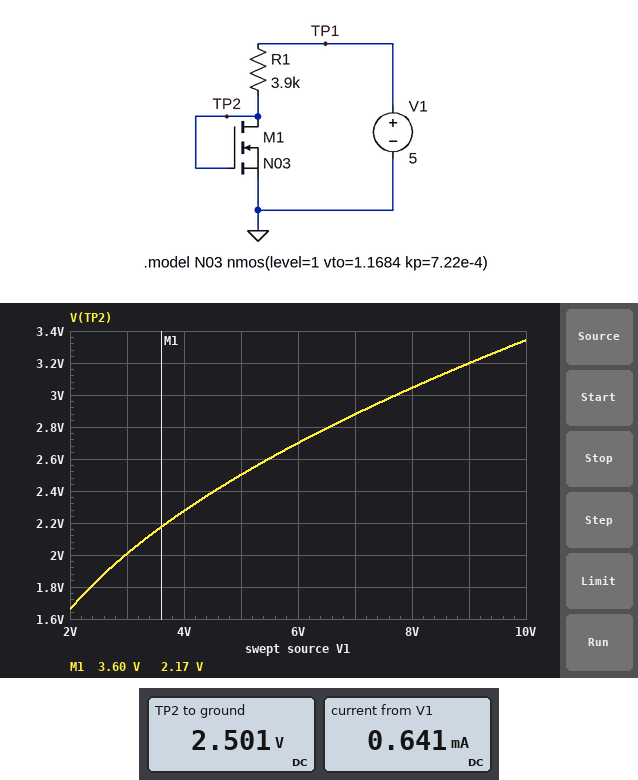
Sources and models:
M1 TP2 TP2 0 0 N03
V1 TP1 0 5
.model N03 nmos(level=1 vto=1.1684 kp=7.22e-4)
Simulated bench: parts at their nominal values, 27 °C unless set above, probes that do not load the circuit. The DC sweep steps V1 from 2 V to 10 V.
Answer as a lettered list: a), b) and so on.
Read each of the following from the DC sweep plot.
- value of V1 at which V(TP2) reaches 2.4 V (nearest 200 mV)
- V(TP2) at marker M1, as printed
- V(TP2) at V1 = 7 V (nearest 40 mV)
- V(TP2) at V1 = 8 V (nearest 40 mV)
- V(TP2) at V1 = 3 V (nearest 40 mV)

a) 4.6 V
b) 2.17 V
c) 2.88 V
d) 3.04 V
e) 2.00 V
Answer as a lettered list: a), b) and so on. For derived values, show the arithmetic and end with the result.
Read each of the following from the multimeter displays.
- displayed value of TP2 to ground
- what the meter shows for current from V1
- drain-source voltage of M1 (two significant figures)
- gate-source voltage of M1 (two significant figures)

a) 2.501 V
b) 0.641 mA
c) 2.501 V = 2.5 V
d) 2.501 V = 2.5 V
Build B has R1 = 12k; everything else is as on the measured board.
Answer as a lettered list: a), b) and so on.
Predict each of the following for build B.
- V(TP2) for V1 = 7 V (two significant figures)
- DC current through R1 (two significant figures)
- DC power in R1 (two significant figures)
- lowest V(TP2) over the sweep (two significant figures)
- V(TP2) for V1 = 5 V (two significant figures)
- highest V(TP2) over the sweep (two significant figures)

a) 2.2 V
b) 250 µA
c) 750 µW
d) 1.5 V
e) 2.0 V
f) 2.5 V
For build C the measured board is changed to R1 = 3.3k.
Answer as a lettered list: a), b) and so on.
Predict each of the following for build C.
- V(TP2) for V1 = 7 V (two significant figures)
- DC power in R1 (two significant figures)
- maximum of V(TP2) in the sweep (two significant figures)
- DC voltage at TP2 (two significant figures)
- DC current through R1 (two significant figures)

a) 3.0 V
b) 1.8 mW
c) 3.5 V
d) 2.6 V
e) 730 µA
